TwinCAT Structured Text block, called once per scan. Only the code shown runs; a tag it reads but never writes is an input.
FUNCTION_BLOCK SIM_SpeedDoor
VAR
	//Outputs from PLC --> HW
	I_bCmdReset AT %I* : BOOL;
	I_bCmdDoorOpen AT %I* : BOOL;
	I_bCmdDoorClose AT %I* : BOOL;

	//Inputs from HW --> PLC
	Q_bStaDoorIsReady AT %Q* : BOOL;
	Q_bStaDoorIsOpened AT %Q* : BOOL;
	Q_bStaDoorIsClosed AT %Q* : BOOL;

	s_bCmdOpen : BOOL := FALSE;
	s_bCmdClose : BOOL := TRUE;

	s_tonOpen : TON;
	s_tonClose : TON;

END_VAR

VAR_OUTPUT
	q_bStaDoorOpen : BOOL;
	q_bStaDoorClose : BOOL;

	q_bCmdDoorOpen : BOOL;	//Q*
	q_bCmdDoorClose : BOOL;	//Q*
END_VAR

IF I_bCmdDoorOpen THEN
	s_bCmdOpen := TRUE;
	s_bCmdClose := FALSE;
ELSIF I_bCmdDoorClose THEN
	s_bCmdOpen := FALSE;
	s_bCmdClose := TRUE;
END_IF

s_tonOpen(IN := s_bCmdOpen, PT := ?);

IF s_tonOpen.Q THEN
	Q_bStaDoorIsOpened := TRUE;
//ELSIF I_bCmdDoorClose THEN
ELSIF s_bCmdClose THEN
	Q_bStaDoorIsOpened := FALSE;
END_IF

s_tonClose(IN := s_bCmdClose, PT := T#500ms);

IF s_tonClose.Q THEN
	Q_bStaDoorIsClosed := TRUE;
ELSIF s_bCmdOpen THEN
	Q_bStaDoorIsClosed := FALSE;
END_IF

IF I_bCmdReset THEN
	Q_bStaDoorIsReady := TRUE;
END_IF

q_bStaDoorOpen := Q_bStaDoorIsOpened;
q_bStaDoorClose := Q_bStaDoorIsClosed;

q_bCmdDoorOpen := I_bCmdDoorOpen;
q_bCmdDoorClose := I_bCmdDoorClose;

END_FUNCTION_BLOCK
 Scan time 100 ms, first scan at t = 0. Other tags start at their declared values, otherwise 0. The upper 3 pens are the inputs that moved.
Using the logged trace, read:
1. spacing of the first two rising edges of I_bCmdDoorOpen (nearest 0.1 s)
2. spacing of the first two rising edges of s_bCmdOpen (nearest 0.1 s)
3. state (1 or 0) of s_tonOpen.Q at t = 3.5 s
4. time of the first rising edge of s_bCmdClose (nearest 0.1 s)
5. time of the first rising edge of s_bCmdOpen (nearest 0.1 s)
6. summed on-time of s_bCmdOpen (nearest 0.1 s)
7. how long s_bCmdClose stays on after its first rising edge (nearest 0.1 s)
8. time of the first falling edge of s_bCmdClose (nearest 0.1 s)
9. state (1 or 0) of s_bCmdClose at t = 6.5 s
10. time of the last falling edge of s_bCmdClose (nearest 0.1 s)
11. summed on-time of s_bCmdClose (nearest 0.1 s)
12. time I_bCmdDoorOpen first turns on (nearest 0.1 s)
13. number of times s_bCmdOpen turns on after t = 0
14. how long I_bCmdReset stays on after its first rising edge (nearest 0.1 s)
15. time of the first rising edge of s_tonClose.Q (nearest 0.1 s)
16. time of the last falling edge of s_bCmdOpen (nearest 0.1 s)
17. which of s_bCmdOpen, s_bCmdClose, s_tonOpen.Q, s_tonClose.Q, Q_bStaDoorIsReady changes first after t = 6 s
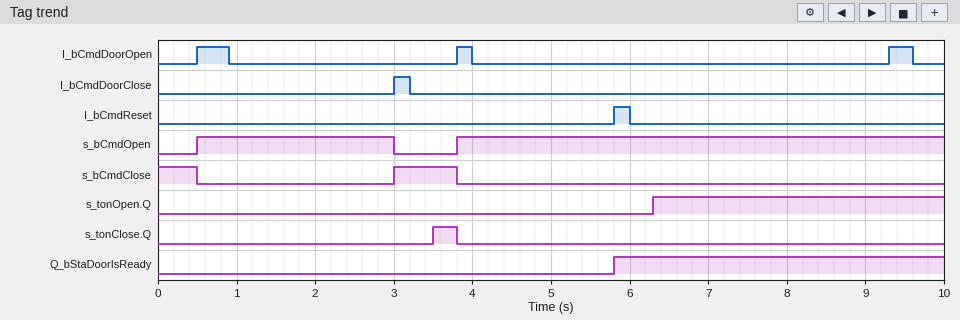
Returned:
3.3 s
3.3 s
0
3.0 s
0.5 s
8.7 s
0.8 s
0.5 s
0
3.8 s
1.3 s
0.5 s
2
0.2 s
3.5 s
3.0 s
s_tonOpen.Q
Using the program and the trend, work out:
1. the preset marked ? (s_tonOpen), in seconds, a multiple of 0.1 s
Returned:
2.5 s
